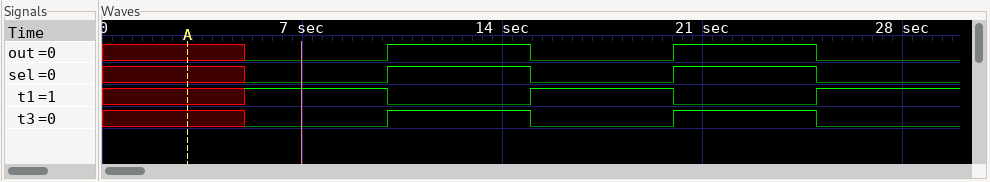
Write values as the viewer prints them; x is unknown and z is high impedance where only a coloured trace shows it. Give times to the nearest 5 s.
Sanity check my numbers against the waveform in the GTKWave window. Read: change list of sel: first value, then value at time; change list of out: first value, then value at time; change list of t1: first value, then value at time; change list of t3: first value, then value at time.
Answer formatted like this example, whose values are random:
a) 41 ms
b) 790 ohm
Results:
a) x, 0 at 5 s, 1 at 10 s, 0 at 15 s, 1 at 20 s, 0 at 25 s
b) x, 0 at 5 s, 1 at 10 s, 0 at 15 s, 1 at 20 s, 0 at 25 s
c) x, 1 at 5 s, 0 at 10 s, 1 at 15 s, 0 at 20 s, 1 at 25 s
d) x, 0 at 5 s, 1 at 10 s, 0 at 15 s, 1 at 20 s, 0 at 25 s
